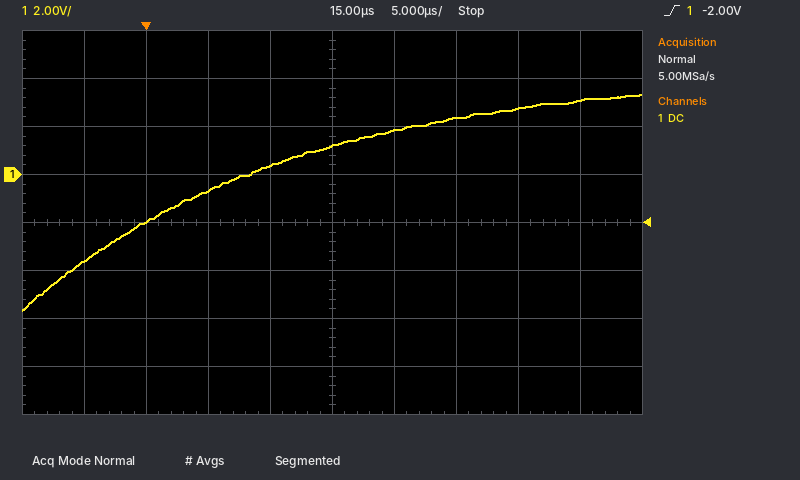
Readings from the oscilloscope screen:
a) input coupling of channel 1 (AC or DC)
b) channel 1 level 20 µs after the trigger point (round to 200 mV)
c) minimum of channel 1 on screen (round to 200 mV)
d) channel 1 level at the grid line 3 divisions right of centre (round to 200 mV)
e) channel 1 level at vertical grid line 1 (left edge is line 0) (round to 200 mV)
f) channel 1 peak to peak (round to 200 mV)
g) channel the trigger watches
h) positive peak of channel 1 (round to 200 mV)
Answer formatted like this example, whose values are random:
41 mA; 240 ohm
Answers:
DC; 1.8 V; -5.6 V; 2.8 V; -3.6 V; 9.0 V; channel 1; 3.4 V
